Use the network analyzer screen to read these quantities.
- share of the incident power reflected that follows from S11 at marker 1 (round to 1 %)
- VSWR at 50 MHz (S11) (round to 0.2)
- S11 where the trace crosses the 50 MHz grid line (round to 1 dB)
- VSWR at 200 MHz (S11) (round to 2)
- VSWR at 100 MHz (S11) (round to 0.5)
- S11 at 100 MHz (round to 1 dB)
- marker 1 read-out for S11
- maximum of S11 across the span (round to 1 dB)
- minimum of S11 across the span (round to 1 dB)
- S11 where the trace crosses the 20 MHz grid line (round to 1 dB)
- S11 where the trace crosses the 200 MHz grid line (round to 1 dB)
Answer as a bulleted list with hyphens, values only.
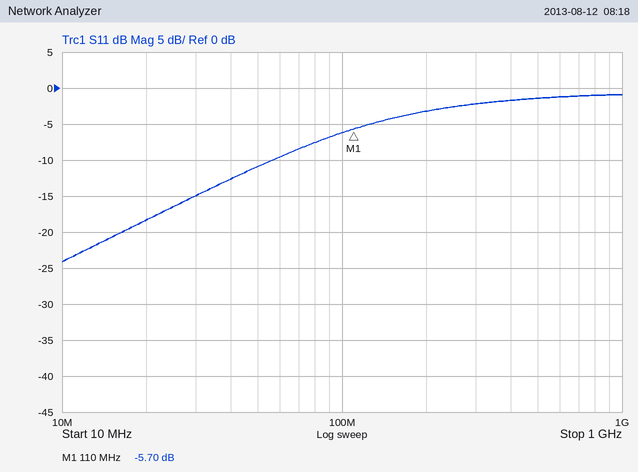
- 27 %
- 1.8
- -11 dB
- 6
- 3.0
- -6 dB
- -5.70 dB
- -1 dB
- -24 dB
- -18 dB
- -3 dB
